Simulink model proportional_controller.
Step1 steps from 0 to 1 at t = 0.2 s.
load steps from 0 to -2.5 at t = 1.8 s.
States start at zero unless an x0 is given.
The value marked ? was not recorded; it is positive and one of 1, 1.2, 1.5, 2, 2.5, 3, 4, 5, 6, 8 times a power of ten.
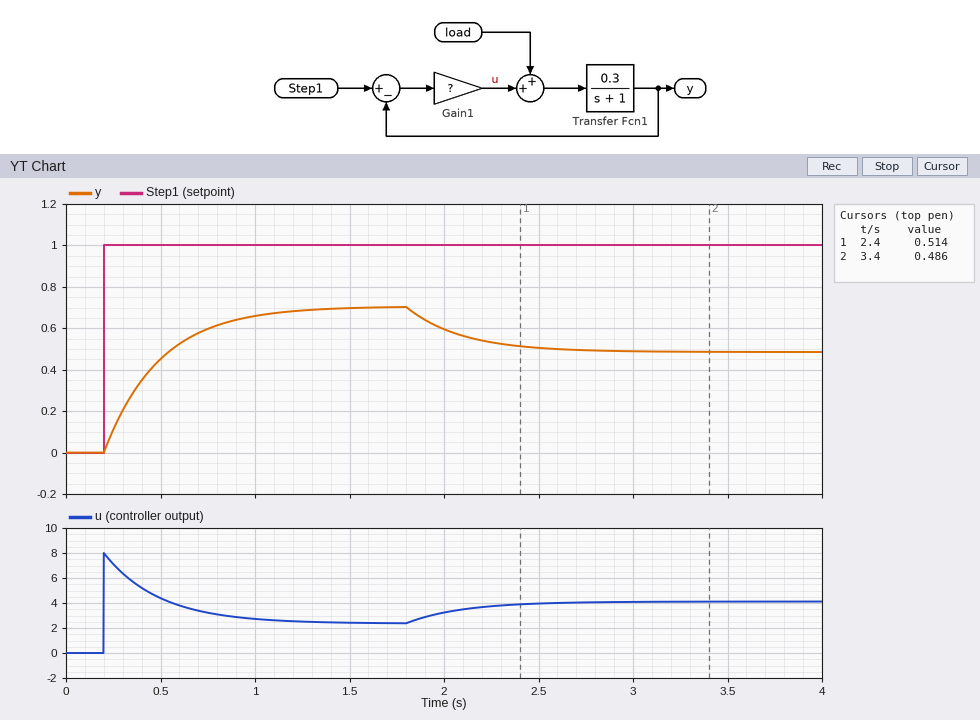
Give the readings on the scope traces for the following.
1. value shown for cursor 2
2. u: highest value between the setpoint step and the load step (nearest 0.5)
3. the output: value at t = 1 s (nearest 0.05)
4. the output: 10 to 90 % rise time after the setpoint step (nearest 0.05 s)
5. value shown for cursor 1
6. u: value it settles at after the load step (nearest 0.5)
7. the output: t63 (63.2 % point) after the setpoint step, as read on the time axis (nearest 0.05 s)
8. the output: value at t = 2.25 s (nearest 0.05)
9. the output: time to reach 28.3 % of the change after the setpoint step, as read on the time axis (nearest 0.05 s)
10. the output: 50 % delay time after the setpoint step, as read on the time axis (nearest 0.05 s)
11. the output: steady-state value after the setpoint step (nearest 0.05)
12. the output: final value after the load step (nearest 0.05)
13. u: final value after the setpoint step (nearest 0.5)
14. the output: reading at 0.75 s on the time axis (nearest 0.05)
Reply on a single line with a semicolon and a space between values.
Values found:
0.486; 8.0; 0.65; 0.65 s; 0.514; 4.0; 0.50 s; 0.55; 0.30 s; 0.40 s; 0.70; 0.50; 2.5; 0.60
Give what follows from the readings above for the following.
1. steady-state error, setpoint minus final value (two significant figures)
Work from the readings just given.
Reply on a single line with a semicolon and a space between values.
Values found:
0.30
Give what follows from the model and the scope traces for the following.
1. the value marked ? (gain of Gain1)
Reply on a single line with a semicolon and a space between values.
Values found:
8
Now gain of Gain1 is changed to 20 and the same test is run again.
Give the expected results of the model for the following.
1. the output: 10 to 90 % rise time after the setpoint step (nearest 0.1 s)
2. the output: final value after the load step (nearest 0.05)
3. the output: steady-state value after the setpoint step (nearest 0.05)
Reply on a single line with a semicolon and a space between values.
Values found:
0.3 s; 0.75; 0.85
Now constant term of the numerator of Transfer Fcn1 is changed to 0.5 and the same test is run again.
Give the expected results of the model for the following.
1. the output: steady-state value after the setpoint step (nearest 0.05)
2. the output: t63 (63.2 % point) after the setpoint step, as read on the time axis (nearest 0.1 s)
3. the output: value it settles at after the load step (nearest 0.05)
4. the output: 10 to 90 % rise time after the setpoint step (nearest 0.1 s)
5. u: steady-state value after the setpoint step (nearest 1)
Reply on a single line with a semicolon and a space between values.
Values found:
0.80; 0.4 s; 0.55; 0.4 s; 2
